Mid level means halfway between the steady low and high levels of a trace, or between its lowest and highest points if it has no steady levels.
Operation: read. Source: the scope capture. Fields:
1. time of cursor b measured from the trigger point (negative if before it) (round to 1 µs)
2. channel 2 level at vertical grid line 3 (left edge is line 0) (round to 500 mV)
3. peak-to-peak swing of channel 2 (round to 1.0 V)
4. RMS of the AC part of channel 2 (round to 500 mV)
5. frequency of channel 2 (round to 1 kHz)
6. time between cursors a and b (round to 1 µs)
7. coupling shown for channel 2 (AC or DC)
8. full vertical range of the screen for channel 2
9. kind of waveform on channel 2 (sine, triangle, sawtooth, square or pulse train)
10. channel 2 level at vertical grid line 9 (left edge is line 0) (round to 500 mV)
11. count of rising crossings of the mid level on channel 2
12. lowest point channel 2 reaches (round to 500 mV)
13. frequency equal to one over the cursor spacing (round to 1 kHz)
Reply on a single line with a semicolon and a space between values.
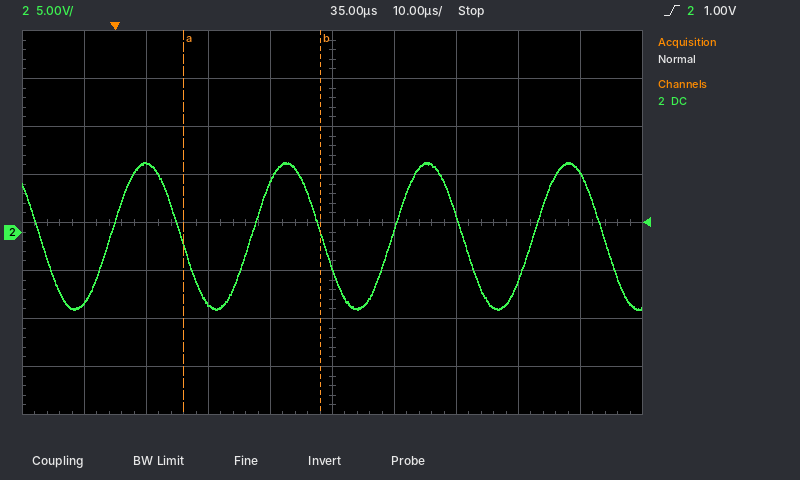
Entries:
+33 µs; -7.5 V; 15.0 V; 5.5 V; 44 kHz; 22 µs; DC; 40 V; sine; 6.0 V; 4; -8.0 V; 45 kHz
